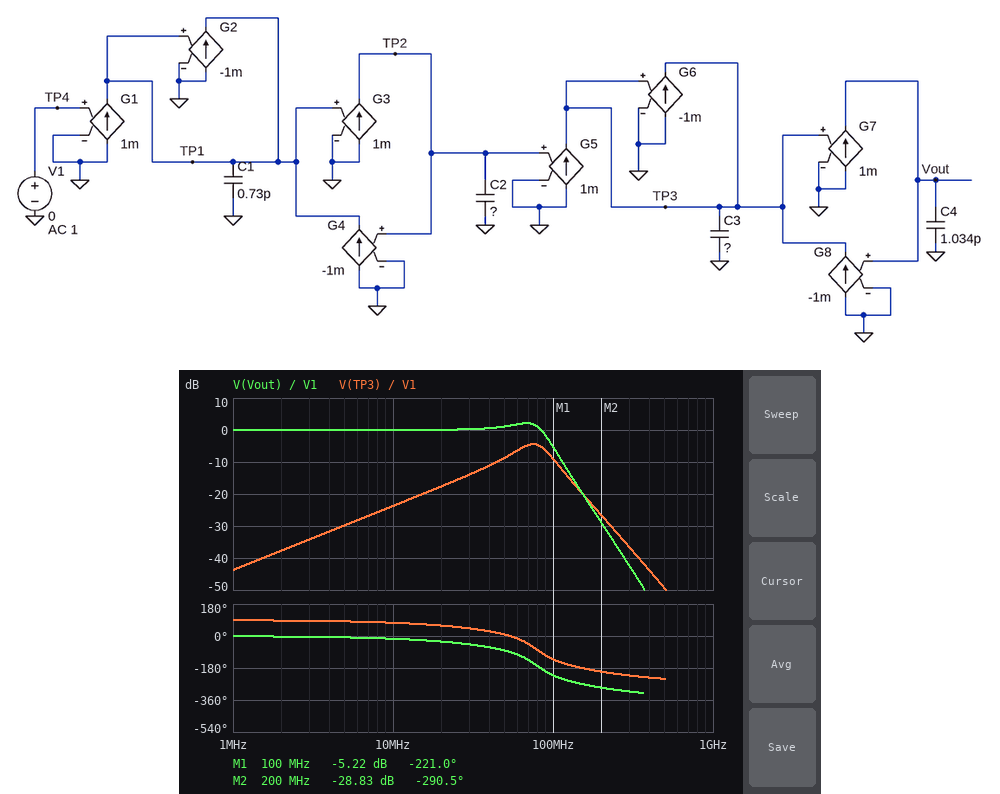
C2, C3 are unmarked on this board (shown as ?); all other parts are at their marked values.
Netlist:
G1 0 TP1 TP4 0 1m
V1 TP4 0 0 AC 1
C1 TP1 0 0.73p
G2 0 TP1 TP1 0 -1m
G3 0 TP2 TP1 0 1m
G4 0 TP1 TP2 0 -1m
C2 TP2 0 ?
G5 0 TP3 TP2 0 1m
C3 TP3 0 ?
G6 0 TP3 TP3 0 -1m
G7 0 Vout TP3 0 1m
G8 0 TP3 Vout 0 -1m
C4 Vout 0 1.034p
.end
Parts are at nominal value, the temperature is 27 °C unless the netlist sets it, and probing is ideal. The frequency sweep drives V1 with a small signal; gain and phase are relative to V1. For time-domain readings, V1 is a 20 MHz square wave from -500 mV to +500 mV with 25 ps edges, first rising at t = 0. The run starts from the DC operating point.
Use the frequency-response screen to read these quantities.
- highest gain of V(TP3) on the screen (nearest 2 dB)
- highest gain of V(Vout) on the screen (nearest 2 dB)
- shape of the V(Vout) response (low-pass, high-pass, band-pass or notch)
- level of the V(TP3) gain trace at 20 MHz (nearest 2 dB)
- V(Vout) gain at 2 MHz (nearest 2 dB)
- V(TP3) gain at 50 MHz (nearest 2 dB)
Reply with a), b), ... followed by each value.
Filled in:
a) -4 dB
b) 2 dB
c) low-pass
d) -18 dB
e) 0 dB
f) -8 dB
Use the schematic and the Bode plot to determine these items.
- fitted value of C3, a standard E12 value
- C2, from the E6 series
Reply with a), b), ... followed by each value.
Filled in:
a) 3.9 pF
b) 3.3 pF
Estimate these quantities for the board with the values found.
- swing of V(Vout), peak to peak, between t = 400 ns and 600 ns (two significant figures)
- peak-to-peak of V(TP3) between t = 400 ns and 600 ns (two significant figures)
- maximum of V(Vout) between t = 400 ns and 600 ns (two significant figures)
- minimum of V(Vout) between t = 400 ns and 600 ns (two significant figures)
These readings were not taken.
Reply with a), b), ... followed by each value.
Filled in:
a) 1.4 V
b) 470 mV
c) 700 mV
d) -700 mV
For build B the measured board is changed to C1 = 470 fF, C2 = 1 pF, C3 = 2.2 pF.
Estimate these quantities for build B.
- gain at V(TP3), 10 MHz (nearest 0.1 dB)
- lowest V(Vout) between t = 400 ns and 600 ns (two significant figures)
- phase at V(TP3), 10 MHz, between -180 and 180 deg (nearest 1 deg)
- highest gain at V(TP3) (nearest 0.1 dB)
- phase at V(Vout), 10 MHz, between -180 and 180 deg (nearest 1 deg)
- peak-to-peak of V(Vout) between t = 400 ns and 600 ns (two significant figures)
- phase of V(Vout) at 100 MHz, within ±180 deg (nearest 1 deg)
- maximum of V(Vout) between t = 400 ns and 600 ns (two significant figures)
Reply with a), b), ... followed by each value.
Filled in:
a) -23.7 dB
b) -820 mV
c) 83 deg
d) -0.3 dB
e) -7 deg
f) 1.6 V
g) -119 deg
h) 820 mV
